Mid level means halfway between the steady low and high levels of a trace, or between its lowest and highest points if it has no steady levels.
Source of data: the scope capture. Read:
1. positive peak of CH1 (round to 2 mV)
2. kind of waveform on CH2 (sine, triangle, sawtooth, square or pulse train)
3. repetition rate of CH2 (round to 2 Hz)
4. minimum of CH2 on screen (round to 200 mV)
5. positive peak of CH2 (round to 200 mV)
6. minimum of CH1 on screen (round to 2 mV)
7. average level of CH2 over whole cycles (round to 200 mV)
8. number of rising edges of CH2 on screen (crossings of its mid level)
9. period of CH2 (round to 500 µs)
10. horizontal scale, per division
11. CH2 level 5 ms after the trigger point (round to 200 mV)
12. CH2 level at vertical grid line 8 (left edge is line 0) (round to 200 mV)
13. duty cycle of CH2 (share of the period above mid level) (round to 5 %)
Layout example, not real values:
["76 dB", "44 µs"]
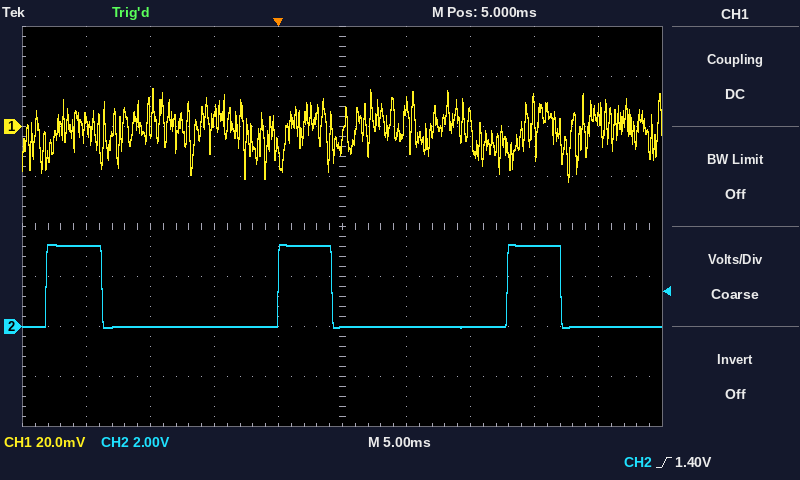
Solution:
["16 mV", "pulse train", "56 Hz", "0.0 V", "3.2 V", "-22 mV", "800 mV", "3", "18.0 ms", "5 ms", "0.0 V", "3.2 V", "25 %"]
